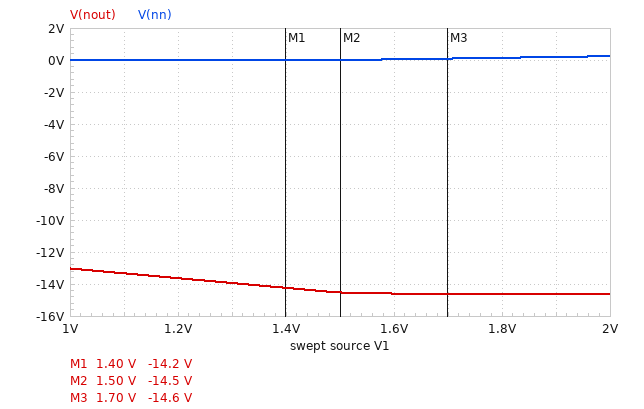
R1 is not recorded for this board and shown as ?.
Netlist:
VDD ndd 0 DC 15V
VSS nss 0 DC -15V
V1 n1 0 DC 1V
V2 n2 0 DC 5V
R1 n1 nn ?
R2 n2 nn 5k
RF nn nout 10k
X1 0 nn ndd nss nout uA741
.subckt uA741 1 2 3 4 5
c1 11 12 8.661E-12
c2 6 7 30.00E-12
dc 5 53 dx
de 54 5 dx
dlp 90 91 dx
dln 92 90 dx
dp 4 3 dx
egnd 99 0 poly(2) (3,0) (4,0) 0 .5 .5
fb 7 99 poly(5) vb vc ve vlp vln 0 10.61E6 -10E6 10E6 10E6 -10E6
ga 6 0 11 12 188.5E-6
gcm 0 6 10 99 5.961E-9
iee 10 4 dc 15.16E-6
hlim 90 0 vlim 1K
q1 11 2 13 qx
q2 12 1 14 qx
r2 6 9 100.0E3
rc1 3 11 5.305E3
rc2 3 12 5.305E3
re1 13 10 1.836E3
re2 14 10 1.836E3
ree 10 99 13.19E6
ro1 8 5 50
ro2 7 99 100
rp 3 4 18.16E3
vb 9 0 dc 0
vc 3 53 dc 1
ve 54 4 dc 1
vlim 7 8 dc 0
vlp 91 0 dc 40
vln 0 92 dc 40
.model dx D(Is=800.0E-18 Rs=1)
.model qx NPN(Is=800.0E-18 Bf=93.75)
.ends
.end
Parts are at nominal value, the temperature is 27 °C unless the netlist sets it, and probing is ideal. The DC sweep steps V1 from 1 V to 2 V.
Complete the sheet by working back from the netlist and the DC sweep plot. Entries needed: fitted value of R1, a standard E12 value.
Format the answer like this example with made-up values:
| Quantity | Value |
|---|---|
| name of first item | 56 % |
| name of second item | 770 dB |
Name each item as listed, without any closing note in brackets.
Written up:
| Quantity | Value |
|---|---|
| fitted value of R1, a standard E12 value | 3.3 kΩ |
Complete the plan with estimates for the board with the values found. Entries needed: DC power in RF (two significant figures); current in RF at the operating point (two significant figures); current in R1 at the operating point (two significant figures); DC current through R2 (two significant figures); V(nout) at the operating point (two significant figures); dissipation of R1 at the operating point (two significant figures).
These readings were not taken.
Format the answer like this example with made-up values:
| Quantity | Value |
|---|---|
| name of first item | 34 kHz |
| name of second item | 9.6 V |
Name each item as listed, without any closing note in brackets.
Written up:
| Quantity | Value |
|---|---|
| DC power in RF | 17 mW |
| current in RF at the operating point | 1.3 mA |
| current in R1 at the operating point | 300 µA |
| DC current through R2 | 1.0 mA |
| V(nout) at the operating point | -13 V |
| dissipation of R1 at the operating point | 300 µW |
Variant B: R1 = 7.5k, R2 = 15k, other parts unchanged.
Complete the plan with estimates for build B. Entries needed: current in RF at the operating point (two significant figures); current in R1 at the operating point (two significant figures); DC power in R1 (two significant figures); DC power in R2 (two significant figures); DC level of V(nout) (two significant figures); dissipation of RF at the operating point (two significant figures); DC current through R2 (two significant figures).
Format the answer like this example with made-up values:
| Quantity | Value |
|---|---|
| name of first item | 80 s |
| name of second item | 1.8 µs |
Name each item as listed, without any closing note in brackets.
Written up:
| Quantity | Value |
|---|---|
| current in RF at the operating point | 470 µA |
| current in R1 at the operating point | 130 µA |
| DC power in R1 | 130 µW |
| DC power in R2 | 1.7 mW |
| DC level of V(nout) | -4.7 V |
| dissipation of RF at the operating point | 2.2 mW |
| DC current through R2 | 330 µA |
